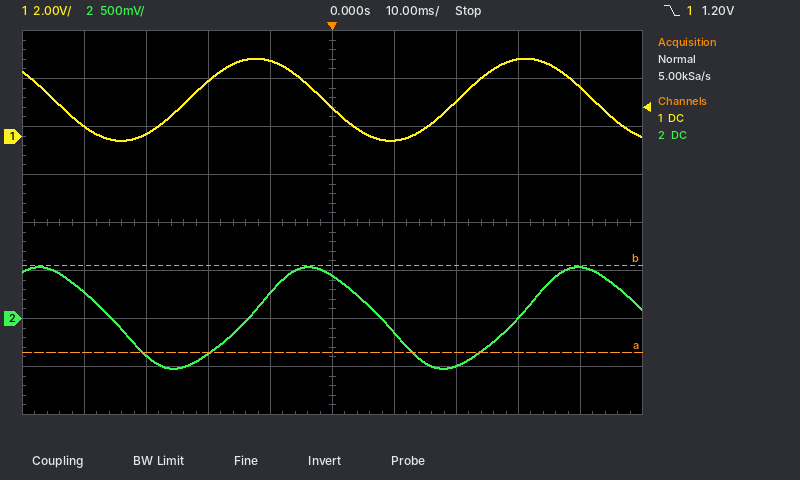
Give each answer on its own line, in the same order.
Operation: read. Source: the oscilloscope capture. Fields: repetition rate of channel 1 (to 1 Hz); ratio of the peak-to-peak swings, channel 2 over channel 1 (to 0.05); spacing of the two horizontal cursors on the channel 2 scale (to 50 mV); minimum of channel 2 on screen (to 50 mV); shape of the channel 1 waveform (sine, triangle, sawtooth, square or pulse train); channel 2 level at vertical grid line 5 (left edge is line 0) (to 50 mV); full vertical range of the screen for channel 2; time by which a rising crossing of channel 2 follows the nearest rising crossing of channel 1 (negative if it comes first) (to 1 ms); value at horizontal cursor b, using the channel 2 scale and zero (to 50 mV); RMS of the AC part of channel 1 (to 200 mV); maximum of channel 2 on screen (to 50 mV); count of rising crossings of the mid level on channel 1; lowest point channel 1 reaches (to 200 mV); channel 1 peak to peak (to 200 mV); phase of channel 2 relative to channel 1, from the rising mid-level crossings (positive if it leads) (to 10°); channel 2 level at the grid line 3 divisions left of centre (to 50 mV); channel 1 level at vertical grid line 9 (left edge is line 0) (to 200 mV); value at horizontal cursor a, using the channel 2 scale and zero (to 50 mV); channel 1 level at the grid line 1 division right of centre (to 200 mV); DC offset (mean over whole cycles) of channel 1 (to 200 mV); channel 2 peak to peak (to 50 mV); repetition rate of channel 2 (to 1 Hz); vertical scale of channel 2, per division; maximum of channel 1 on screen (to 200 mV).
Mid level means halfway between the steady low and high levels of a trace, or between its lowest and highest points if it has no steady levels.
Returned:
23 Hz
0.30
900 mV
-500 mV
sine
450 mV
4 V
+10 ms
550 mV
1.2 V
550 mV
2
-200 mV
3.4 V
-80°
-400 mV
2.0 V
-350 mV
-200 mV
1.6 V
1.05 V
23 Hz
500 mV
3.2 V
